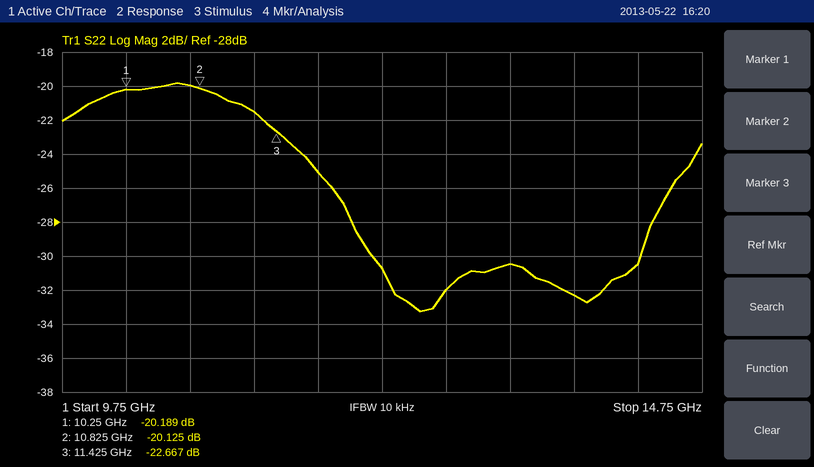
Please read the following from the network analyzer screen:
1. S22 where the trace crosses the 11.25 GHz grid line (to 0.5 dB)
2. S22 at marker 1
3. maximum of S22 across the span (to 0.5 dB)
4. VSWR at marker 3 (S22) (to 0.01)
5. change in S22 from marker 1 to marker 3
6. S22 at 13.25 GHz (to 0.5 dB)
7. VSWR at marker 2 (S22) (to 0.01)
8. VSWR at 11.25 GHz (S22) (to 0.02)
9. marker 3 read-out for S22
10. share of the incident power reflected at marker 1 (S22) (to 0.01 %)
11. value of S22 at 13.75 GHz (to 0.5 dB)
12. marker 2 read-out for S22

-21.5 dB
-20.189 dB
-20.0 dB
1.16
-2.478 dB
-30.5 dB
1.22
1.18
-22.667 dB
0.96 %
-32.5 dB
-20.125 dB
